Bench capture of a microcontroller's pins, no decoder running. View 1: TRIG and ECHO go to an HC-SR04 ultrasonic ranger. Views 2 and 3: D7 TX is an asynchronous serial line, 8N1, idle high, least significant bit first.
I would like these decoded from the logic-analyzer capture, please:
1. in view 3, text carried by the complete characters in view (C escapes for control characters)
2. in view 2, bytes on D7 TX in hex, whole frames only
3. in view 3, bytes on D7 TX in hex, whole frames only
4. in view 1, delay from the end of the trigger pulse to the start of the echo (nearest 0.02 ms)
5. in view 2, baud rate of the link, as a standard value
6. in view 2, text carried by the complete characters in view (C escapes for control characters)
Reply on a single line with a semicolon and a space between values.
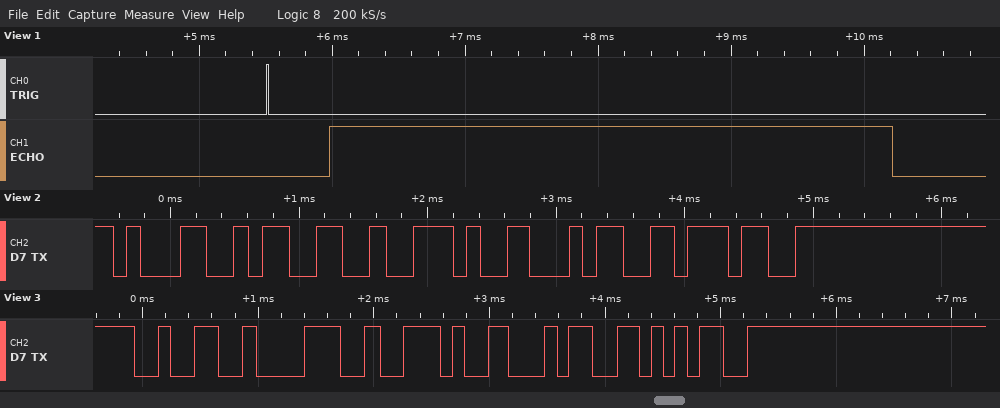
"28.45"; 31 33 2E 34 37; 32 38 2E 34 35; 0.46 ms; 9600 baud; "13.47"
